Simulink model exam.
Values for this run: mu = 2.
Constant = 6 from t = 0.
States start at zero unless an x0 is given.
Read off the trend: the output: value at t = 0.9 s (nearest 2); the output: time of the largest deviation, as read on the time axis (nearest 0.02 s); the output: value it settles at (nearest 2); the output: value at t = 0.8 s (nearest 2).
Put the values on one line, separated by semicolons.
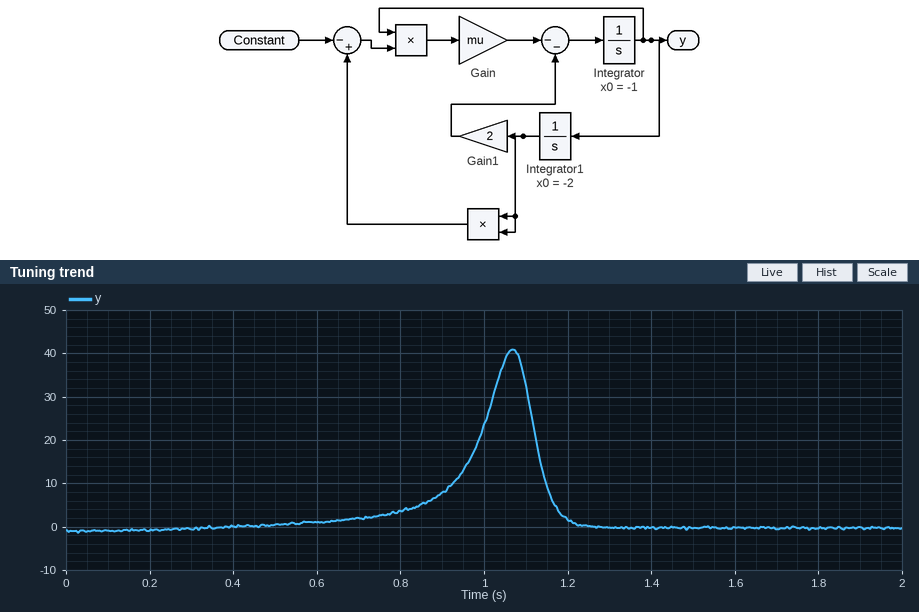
8; 1.06 s; 0; 4
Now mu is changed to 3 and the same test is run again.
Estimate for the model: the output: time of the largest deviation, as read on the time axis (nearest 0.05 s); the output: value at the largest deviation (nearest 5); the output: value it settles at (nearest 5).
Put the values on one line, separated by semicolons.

1.15 s; 60; 0
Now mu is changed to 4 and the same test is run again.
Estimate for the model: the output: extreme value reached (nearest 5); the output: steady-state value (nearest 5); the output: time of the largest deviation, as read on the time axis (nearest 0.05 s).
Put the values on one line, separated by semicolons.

80; 0; 1.25 s
